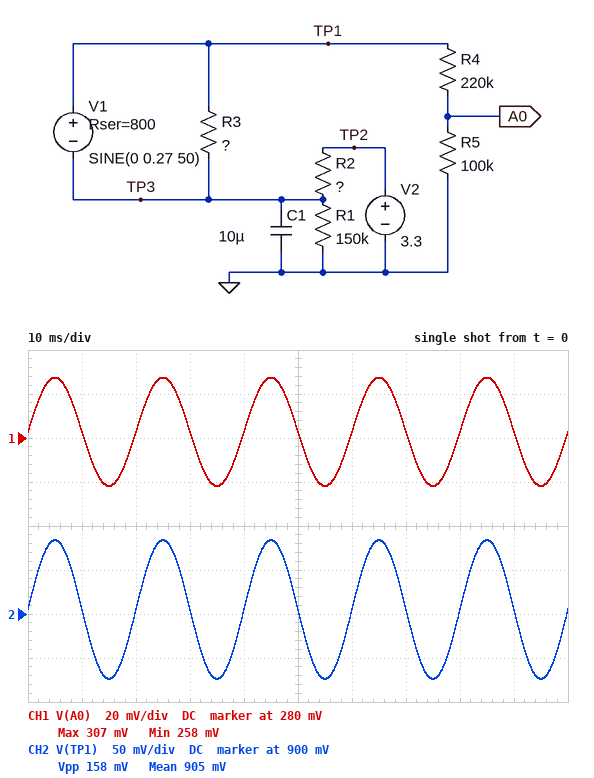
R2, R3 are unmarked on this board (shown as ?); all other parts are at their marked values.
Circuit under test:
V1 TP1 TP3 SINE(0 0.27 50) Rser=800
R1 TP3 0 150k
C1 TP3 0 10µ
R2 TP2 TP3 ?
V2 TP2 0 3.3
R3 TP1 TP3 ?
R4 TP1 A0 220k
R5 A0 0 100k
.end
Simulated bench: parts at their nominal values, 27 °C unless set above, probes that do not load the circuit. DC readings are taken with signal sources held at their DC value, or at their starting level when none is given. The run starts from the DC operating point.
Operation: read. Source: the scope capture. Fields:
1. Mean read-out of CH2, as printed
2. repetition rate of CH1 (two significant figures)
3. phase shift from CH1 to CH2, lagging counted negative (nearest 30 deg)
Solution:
905 mV
50 Hz
0 deg
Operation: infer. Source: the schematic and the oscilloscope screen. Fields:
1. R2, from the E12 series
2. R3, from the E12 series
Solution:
270 kΩ
330 Ω
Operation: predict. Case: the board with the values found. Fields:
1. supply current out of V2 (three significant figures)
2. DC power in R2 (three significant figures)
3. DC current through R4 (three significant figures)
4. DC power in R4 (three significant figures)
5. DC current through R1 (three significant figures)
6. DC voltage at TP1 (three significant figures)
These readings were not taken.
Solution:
8.87 µA
21.2 µW
2.83 µA
1.76 µW
6.04 µA
905 mV
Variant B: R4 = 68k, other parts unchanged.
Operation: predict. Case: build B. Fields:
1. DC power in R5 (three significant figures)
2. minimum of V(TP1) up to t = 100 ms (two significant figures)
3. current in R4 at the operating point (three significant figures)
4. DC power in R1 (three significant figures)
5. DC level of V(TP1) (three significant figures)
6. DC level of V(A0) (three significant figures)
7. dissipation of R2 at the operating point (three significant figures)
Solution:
1.98 µW
670 mV
4.45 µA
3.74 µW
748 mV
445 mV
24.1 µW
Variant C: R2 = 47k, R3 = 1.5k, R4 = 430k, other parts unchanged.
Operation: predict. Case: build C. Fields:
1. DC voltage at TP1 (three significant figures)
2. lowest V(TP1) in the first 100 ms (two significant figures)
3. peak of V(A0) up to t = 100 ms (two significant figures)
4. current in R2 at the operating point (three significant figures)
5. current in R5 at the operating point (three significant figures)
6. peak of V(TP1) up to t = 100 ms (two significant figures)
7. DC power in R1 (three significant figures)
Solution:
2.35 V
2.2 V
480 mV
20.1 µA
4.44 µA
2.5 V
36.9 µW
